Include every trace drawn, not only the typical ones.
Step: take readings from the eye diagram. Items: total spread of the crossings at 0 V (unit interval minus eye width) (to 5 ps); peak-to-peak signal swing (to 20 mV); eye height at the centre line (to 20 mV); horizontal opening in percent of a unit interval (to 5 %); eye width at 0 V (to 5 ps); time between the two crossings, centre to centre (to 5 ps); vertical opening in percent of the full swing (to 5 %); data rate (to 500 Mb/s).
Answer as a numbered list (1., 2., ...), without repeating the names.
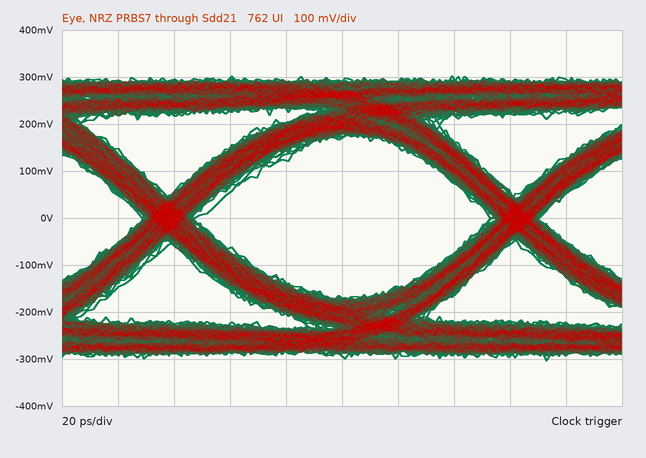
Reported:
1. 20 ps
2. 600 mV
3. 340 mV
4. 85 %
5. 105 ps
6. 125 ps
7. 55 %
8. 8.0 Gb/s
